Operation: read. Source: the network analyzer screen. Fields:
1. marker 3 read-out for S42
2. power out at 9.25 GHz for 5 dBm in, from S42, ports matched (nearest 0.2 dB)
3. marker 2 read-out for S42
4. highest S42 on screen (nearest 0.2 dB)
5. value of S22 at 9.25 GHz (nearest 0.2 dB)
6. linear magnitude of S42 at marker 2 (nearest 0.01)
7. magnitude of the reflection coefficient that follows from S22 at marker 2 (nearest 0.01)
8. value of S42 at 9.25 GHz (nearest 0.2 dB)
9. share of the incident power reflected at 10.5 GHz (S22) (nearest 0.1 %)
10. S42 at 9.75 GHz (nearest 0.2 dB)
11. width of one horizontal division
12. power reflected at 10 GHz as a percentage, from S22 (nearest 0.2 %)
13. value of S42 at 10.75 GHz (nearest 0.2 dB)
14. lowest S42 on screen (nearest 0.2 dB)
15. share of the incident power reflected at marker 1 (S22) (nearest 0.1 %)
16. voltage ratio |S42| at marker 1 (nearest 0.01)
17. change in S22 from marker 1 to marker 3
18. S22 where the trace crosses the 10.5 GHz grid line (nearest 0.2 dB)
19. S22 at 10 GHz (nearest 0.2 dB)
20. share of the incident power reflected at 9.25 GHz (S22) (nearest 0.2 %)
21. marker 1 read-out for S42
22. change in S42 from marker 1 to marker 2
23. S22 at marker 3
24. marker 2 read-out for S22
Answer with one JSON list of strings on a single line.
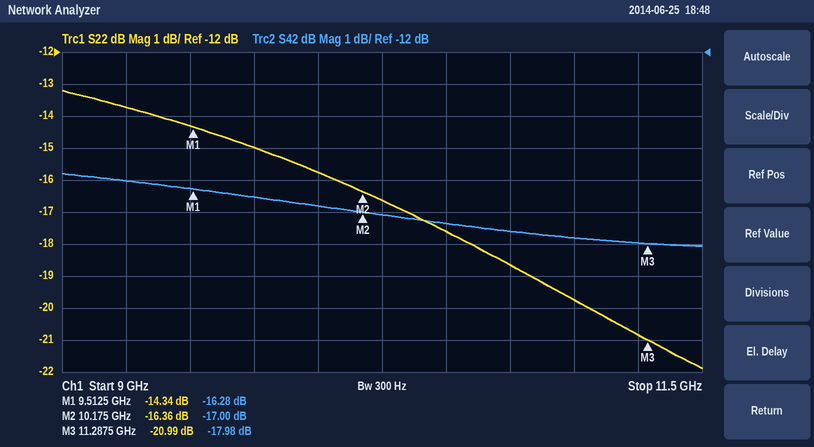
["-17.98 dB", "-11.0 dBm", "-17.00 dB", "-15.8 dB", "-13.8 dB", "0.14", "0.15", "-16.0 dB", "1.7 %", "-16.6 dB", "250 MHz", "2.6 %", "-17.6 dB", "-18.0 dB", "3.7 %", "0.15", "-6.65 dB", "-17.6 dB", "-15.8 dB", "4.2 %", "-16.28 dB", "-0.72 dB", "-20.99 dB", "-16.36 dB"]
